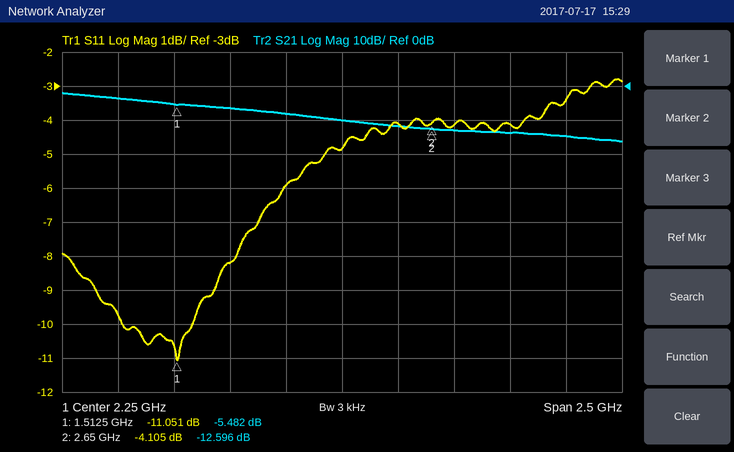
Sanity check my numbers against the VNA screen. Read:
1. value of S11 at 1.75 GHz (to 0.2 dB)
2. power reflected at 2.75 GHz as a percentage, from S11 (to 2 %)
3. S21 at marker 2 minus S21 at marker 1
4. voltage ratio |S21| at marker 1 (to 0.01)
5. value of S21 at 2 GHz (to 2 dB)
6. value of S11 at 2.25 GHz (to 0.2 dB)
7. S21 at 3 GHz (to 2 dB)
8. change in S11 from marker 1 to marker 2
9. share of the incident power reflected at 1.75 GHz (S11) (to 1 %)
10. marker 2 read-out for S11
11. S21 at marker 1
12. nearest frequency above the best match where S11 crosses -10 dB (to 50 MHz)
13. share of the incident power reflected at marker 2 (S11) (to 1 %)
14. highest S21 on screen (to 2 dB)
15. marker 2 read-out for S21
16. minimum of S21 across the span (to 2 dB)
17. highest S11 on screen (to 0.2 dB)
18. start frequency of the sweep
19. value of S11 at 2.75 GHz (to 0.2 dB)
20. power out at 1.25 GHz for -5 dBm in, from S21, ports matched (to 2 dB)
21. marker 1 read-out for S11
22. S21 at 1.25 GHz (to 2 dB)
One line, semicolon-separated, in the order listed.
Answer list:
-8.2 dB; 38 %; -7.114 dB; 0.53; -8 dB; -4.8 dB; -14 dB; 6.946 dB; 15 %; -4.105 dB; -5.482 dB; 1.60 GHz; 39 %; -2 dB; -12.596 dB; -16 dB; -2.8 dB; 1 GHz; -4.2 dB; -8 dBm; -11.051 dB; -4 dB
